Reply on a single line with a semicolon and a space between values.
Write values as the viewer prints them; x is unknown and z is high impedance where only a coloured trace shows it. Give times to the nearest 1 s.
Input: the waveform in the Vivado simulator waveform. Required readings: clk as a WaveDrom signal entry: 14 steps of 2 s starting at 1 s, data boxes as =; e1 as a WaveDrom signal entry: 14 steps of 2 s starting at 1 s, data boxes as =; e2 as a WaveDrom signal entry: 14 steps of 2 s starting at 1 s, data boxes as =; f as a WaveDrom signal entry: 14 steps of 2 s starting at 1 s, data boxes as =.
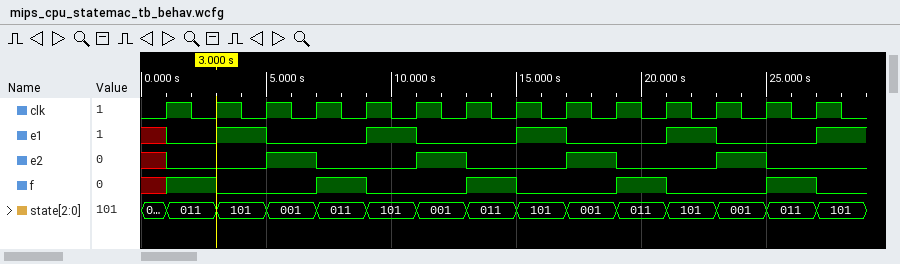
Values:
{name: 'clk', wave: 'p.............'}; {name: 'e1', wave: '010.10.10.10.1'}; {name: 'e2', wave: '0.10.10.10.10.'}; {name: 'f', wave: '10.10.10.10.10'}
